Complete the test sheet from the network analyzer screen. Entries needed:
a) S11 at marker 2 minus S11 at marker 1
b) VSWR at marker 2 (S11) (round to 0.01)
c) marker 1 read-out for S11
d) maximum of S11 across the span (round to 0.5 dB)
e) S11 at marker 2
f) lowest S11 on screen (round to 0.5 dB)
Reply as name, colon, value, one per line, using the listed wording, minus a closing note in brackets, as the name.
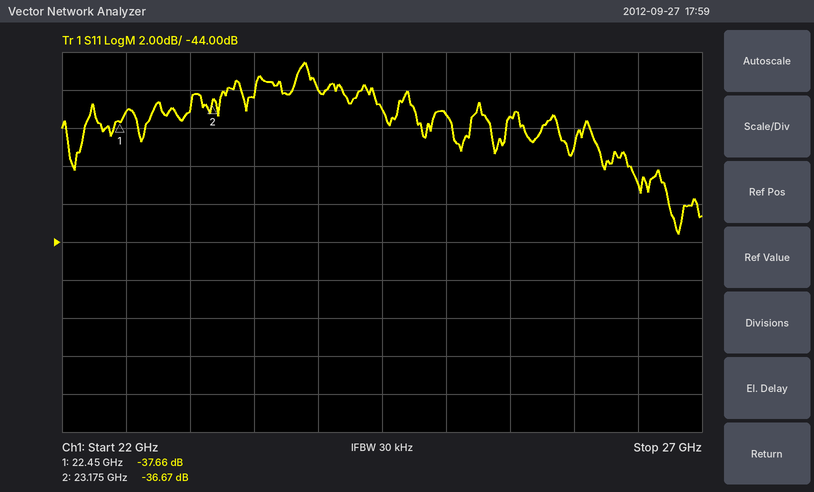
S11 at marker 2 minus S11 at marker 1: 0.99 dB
VSWR at marker 2 (S11): 1.03
marker 1 read-out for S11: -37.66 dB
maximum of S11 across the span: -34.5 dB
S11 at marker 2: -36.67 dB
lowest S11 on screen: -43.5 dB
